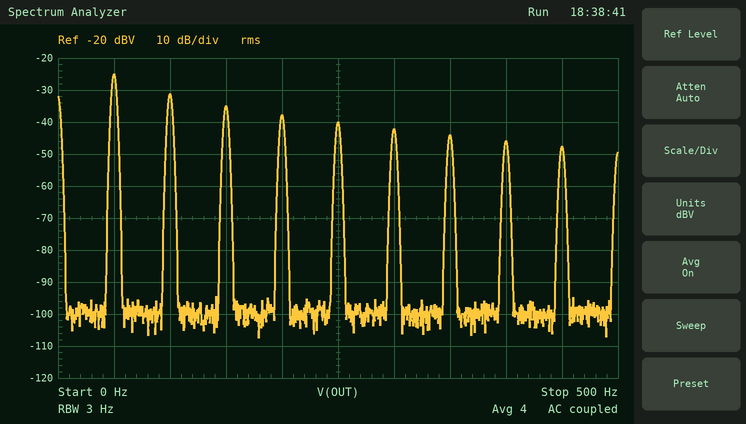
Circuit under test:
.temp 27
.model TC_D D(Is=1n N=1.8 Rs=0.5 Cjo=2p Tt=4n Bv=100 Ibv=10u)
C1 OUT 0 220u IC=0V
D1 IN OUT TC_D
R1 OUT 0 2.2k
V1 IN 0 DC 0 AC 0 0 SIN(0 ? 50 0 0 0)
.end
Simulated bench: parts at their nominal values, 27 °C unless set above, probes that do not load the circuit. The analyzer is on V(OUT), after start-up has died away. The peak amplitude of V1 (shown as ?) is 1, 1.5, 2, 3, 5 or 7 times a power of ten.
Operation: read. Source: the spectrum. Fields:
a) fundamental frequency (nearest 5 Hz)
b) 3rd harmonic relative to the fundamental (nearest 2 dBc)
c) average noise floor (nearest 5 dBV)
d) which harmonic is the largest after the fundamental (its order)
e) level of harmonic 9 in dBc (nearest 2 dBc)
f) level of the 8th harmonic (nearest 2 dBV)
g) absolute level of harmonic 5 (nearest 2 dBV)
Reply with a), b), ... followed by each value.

a) 50 Hz
b) -10 dBc
c) -100 dBV
d) 2
e) -22 dBc
f) -46 dBV
g) -40 dBV
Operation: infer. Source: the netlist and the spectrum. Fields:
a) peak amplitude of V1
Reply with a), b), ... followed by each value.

a) 7 V
